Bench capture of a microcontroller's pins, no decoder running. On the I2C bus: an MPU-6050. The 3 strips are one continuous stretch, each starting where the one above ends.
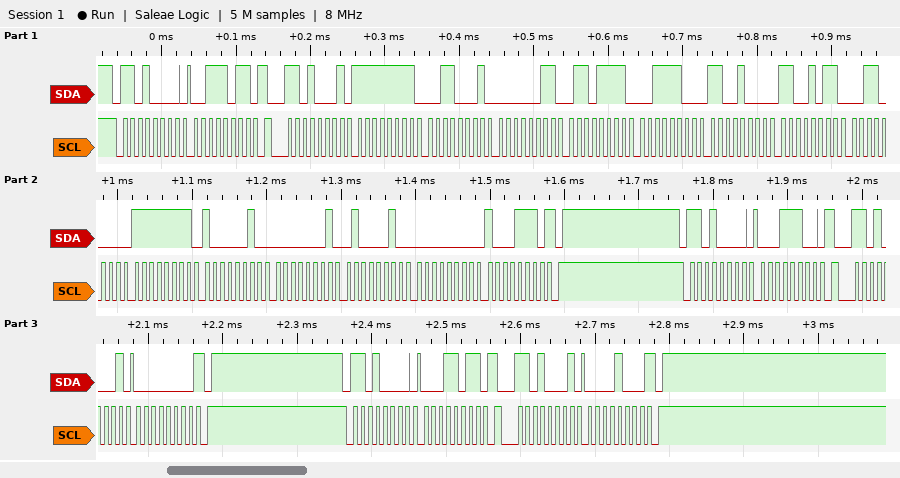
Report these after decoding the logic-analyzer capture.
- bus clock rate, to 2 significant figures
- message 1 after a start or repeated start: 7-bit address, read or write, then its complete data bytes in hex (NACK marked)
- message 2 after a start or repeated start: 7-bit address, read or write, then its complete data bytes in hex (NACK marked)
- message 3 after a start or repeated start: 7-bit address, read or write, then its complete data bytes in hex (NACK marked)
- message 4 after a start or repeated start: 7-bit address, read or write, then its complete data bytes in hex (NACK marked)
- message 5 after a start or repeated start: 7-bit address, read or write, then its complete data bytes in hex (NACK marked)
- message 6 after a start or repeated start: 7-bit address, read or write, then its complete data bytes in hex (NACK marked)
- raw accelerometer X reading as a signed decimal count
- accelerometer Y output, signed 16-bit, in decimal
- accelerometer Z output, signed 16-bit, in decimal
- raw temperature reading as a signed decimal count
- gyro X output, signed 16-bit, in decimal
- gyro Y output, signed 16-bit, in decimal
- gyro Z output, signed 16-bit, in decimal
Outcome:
100 kHz
0x68 write: 3B
0x68 read: FF 31 03 6F 3C C8 CB 30 FF 82 01 42 00 8E NACK
0x68 write: 1C
0x68 read: 00 NACK
0x68 write: 1B
0x68 read: 08 NACK
-207
879
15560
-13520
-126
322
142
